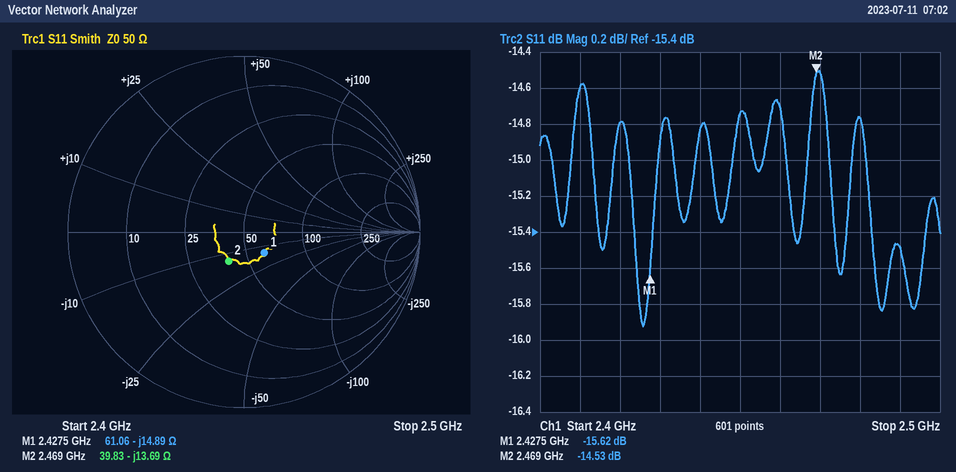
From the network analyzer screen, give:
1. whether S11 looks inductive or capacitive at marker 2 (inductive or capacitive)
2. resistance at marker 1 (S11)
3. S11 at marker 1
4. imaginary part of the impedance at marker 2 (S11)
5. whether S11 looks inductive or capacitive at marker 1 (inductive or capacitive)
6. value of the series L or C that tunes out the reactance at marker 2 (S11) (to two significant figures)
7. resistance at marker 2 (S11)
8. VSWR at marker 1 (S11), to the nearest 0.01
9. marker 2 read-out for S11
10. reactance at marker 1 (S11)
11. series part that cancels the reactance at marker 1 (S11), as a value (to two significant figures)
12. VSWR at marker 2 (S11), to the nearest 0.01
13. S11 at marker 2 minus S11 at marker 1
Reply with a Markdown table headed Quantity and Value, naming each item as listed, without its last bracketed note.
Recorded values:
| Quantity | Value |
|---|---|
| whether S11 looks inductive or capacitive at marker 2 | capacitive |
| resistance at marker 1 | 61.06 Ω |
| S11 at marker 1 | -15.62 dB |
| imaginary part of the impedance at marker 2 | -13.69 Ω |
| whether S11 looks inductive or capacitive at marker 1 | capacitive |
| value of the series L or C that tunes out the reactance at marker 2 (S11) | 880 pH |
| resistance at marker 2 | 39.83 Ω |
| VSWR at marker 1 (S11), to the nearest 0.01 | 1.40 |
| marker 2 read-out for S11 | -14.53 dB |
| reactance at marker 1 | -14.89 Ω |
| series part that cancels the reactance at marker 1 (S11), as a value | 980 pH |
| VSWR at marker 2 (S11), to the nearest 0.01 | 1.46 |
| S11 at marker 2 minus S11 at marker 1 | 1.09 dB |
